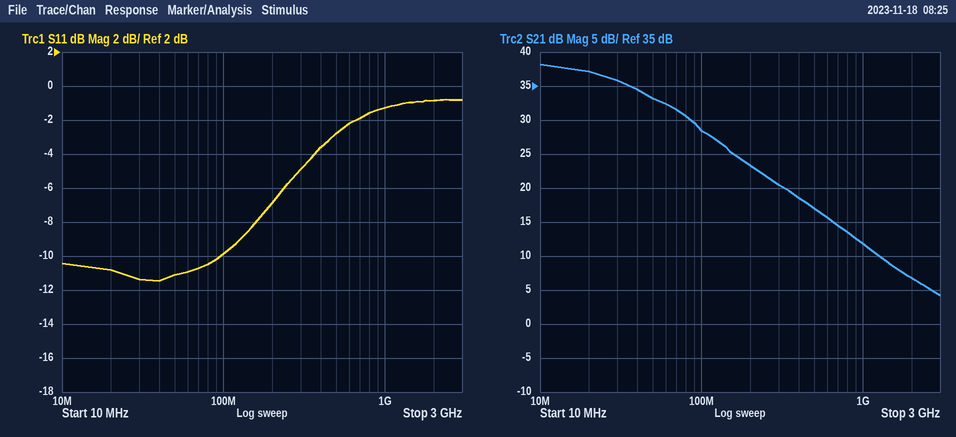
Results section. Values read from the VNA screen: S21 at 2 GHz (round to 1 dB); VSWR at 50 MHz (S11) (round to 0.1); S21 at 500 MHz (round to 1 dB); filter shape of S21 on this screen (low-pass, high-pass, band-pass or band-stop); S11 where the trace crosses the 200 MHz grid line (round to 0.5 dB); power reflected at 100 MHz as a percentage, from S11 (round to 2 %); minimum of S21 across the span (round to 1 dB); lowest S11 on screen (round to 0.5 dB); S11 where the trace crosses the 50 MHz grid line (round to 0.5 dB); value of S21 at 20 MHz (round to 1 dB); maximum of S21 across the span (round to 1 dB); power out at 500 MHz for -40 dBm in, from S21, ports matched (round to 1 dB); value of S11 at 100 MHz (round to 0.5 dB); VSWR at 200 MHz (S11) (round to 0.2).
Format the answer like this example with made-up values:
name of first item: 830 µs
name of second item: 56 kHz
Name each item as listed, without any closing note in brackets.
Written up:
S21 at 2 GHz: 7 dB
VSWR at 50 MHz (S11): 1.8
S21 at 500 MHz: 17 dB
filter shape of S21 on this screen: low-pass
S11 where the trace crosses the 200 MHz grid line: -7.0 dB
power reflected at 100 MHz as a percentage, from S11: 10 %
minimum of S21 across the span: 4 dB
lowest S11 on screen: -11.5 dB
S11 where the trace crosses the 50 MHz grid line: -11.0 dB
value of S21 at 20 MHz: 37 dB
maximum of S21 across the span: 38 dB
power out at 500 MHz for -40 dBm in, from S21, ports matched: -23 dBm
value of S11 at 100 MHz: -10.0 dB
VSWR at 200 MHz (S11): 2.6
